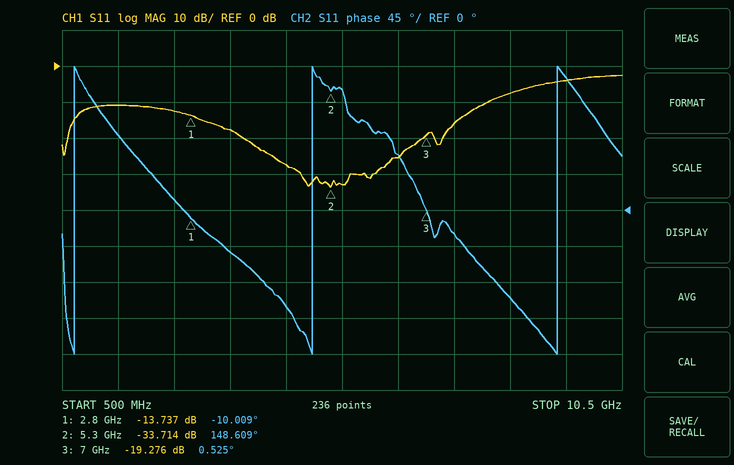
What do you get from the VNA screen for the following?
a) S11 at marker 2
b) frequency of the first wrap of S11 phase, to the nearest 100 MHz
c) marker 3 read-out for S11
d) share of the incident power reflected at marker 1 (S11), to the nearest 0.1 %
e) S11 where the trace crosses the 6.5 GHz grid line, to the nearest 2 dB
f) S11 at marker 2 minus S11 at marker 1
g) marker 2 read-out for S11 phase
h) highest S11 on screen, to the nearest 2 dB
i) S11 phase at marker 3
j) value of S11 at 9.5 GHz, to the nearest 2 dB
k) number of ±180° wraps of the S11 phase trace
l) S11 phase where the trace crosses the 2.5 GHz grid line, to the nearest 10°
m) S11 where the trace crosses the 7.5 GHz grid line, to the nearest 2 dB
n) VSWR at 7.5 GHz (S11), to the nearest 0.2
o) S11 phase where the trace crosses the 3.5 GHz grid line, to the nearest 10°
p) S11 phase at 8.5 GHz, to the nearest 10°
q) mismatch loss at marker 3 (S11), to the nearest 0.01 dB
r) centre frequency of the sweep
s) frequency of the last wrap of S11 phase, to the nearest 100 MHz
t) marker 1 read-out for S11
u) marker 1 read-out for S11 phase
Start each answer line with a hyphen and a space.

- -33.714 dB
- 700 MHz
- -19.276 dB
- 4.2 %
- -26 dB
- -19.977 dB
- 148.609°
- -2 dB
- 0.525°
- -4 dB
- 3
- 10°
- -16 dB
- 1.4
- -50°
- -110°
- 0.05 dB
- 5.5 GHz
- 9.3 GHz
- -13.737 dB
- -10.009°
